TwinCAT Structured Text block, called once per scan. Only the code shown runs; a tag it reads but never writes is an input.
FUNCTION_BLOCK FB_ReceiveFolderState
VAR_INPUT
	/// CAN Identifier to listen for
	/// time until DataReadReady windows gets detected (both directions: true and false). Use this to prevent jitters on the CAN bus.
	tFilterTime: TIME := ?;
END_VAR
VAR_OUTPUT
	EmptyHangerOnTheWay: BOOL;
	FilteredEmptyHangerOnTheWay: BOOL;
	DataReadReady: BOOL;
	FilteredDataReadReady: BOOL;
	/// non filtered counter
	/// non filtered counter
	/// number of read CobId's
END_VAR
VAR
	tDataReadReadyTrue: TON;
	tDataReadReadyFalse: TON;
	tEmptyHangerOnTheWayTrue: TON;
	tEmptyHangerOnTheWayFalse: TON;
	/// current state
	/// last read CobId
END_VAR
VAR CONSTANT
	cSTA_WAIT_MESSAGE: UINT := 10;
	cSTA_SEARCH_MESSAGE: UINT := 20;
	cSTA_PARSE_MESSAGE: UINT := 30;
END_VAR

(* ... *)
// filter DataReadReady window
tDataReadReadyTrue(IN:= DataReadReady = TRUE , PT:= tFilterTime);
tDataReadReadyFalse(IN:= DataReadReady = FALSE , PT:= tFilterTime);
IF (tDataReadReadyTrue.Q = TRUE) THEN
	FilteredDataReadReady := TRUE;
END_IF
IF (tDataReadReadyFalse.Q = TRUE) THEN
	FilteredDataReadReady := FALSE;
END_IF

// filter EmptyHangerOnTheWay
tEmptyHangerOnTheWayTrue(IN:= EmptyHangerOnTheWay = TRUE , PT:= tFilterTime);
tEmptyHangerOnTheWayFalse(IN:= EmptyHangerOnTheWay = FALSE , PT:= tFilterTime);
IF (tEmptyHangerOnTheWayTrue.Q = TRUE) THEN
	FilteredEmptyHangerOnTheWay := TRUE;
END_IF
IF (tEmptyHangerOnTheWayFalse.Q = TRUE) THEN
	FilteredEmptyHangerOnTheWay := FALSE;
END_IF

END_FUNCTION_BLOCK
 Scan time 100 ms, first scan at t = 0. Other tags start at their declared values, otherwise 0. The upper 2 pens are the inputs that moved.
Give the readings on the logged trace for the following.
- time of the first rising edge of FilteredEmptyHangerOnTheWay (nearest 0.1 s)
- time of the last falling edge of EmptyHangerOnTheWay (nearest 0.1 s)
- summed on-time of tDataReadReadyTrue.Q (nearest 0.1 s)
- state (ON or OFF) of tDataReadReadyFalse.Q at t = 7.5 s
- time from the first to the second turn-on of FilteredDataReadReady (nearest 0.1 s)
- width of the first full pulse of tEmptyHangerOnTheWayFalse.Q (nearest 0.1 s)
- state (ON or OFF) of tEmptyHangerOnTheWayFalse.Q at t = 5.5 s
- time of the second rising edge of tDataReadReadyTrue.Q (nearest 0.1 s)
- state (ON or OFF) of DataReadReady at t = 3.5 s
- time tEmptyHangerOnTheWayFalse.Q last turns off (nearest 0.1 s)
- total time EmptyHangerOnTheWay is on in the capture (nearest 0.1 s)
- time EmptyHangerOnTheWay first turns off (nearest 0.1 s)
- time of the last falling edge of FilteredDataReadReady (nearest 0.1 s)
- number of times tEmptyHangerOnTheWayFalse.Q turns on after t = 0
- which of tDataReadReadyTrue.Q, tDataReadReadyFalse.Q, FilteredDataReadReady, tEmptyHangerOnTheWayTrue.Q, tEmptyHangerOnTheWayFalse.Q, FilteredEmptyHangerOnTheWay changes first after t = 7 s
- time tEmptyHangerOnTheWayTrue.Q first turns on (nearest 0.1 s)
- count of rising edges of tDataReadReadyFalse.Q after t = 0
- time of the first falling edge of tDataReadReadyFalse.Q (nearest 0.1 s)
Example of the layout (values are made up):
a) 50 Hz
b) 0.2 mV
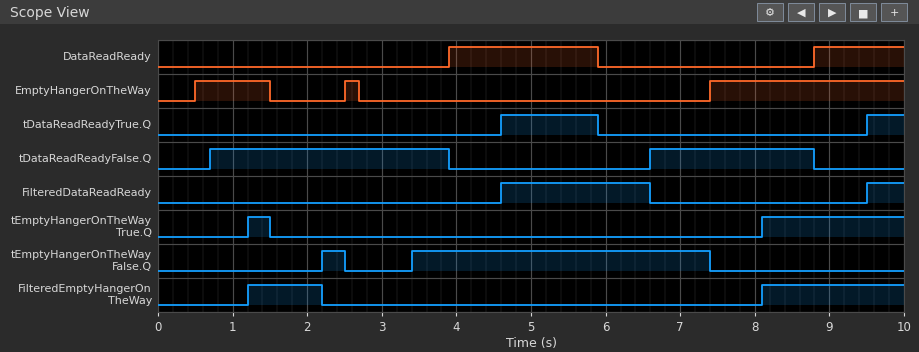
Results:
a) 1.2 s
b) 2.7 s
c) 1.8 s
d) ON
e) 4.9 s
f) 0.3 s
g) ON
h) 9.5 s
i) OFF
j) 7.4 s
k) 3.8 s
l) 1.5 s
m) 6.6 s
n) 2
o) tEmptyHangerOnTheWayFalse.Q
p) 1.2 s
q) 2
r) 3.9 s
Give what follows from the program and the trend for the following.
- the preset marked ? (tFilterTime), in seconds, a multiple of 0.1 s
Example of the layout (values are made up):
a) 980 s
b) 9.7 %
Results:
a) 0.7 s
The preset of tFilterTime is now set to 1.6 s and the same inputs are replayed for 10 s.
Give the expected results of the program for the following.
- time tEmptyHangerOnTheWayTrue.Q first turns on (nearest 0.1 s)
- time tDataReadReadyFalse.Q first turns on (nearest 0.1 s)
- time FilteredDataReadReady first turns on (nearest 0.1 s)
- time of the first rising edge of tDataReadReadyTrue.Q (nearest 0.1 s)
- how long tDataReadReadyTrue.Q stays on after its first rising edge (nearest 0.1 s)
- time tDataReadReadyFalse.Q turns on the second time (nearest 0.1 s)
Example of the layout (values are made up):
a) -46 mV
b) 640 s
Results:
a) 9.0 s
b) 1.6 s
c) 5.5 s
d) 5.5 s
e) 0.4 s
f) 7.5 s
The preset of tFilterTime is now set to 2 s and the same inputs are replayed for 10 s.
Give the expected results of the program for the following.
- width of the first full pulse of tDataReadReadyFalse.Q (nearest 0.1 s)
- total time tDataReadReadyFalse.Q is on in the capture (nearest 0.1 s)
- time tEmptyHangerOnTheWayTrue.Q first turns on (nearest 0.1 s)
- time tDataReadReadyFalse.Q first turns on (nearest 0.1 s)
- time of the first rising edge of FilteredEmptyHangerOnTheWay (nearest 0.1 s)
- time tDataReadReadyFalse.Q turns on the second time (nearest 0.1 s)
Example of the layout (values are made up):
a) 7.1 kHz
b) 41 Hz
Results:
a) 1.9 s
b) 2.8 s
c) 9.4 s
d) 2.0 s
e) 9.4 s
f) 7.9 s
